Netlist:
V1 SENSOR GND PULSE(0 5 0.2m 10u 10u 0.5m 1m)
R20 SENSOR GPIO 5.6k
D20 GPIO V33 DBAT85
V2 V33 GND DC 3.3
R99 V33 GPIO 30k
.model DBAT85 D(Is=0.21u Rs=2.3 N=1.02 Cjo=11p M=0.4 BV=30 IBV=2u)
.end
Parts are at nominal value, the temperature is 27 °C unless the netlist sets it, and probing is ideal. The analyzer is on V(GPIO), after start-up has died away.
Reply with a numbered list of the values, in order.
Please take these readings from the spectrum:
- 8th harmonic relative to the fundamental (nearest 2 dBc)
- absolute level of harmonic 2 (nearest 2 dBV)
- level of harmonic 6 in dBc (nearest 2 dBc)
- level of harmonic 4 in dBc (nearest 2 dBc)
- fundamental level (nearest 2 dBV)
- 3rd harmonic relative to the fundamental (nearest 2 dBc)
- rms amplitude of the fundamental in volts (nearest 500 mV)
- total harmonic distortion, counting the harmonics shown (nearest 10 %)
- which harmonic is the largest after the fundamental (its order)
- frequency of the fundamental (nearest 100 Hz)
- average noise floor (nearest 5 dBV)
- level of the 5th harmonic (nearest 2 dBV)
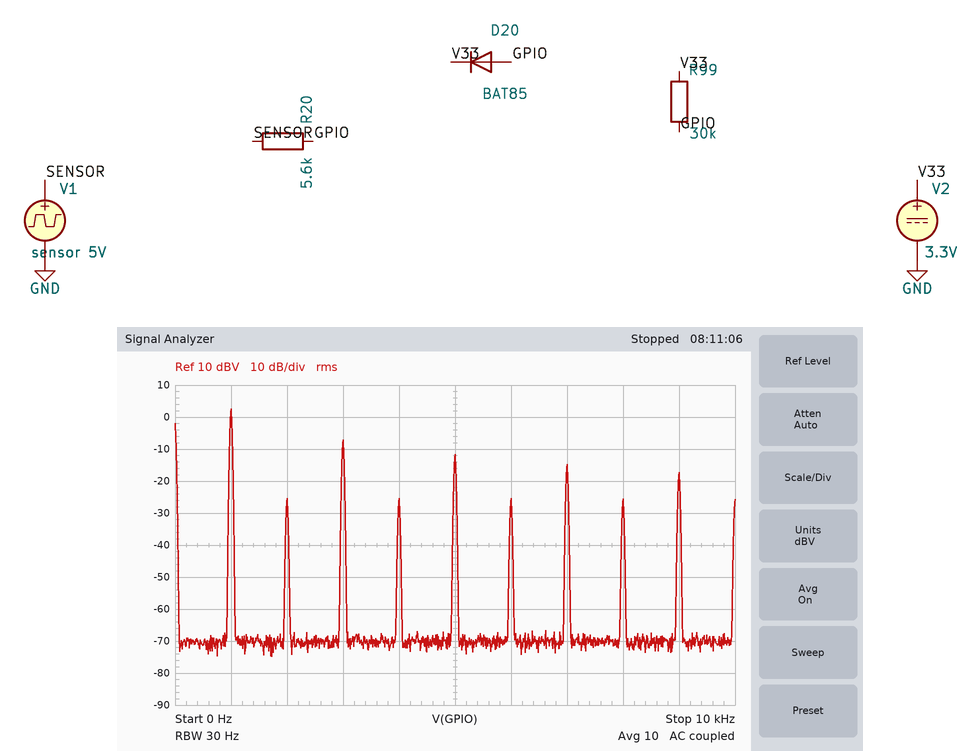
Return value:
1. -28 dBc
2. -26 dBV
3. -28 dBc
4. -28 dBc
5. 2 dBV
6. -10 dBc
7. 1.5 V
8. 40 %
9. 3
10. 1.0 kHz
11. -70 dBV
12. -12 dBV
